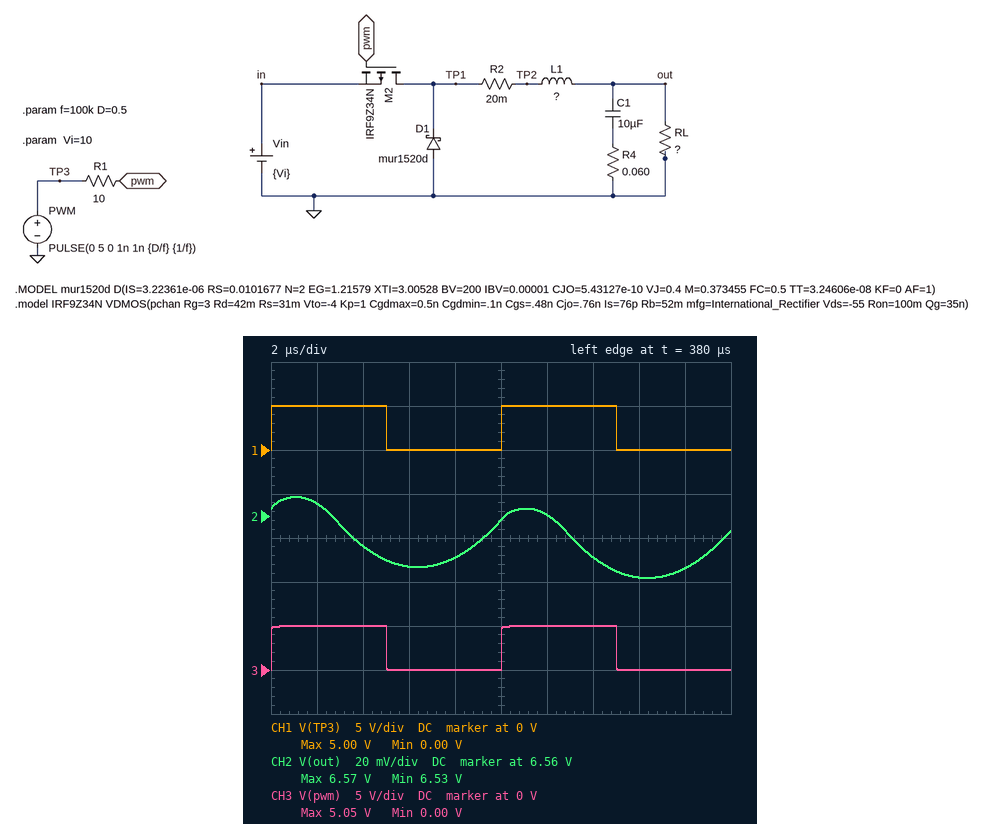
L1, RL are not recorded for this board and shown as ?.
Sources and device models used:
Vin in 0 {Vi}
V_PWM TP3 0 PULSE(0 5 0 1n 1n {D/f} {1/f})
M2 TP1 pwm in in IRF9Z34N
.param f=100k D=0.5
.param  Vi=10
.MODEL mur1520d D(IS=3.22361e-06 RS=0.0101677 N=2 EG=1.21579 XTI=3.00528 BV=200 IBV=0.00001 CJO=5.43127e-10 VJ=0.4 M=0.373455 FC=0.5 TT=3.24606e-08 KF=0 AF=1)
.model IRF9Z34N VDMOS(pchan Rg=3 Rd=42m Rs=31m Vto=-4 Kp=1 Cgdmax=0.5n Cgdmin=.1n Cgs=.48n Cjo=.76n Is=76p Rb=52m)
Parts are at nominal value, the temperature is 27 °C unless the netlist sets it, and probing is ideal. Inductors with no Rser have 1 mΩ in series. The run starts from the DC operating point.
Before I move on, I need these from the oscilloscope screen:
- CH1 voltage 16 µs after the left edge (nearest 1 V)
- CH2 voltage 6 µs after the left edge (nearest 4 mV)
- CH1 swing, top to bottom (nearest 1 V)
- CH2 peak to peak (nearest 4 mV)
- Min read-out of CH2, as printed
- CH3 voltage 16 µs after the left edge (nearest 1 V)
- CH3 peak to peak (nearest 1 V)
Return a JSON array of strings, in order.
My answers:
["0 V", "6.536 V", "5 V", "36 mV", "6.53 V", "0 V", "5 V"]
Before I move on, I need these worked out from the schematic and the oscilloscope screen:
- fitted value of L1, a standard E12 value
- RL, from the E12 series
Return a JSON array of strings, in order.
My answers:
["100 µH", "12 Ω"]
